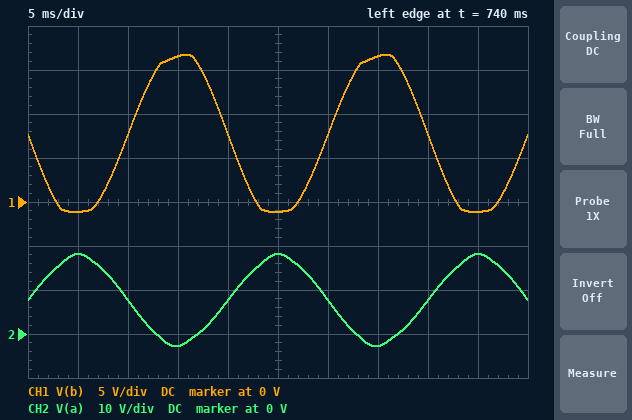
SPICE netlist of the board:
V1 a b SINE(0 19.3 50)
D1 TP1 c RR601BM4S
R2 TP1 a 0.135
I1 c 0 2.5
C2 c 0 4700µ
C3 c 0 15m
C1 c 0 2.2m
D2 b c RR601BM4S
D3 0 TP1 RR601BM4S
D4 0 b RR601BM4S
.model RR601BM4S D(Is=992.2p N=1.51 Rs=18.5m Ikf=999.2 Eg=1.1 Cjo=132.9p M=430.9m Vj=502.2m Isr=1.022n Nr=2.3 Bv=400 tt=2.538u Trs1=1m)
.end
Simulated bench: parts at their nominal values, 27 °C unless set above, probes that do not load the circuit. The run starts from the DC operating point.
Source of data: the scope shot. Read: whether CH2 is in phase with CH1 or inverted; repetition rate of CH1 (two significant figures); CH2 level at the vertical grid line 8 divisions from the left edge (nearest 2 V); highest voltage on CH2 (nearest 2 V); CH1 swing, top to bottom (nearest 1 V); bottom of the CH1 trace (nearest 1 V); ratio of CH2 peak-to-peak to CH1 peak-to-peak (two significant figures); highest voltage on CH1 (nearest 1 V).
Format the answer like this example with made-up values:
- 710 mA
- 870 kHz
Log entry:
- inverted
- 50 Hz
- 8 V
- 18 V
- 18 V
- -1 V
- 1.2
- 17 V
